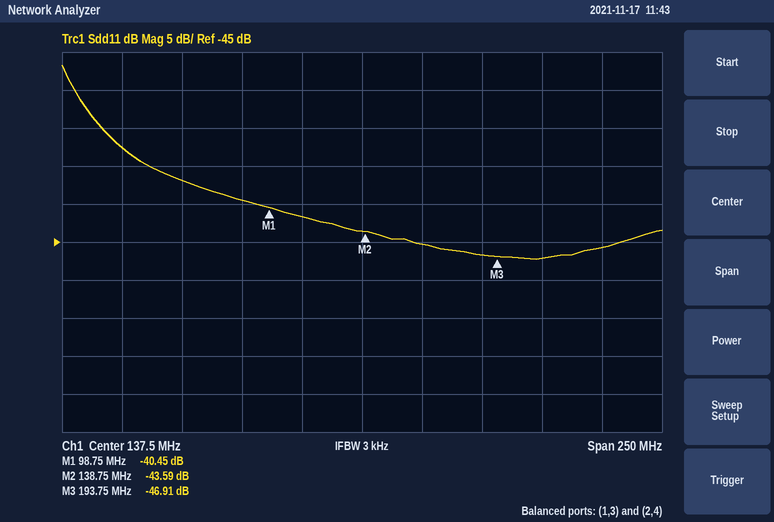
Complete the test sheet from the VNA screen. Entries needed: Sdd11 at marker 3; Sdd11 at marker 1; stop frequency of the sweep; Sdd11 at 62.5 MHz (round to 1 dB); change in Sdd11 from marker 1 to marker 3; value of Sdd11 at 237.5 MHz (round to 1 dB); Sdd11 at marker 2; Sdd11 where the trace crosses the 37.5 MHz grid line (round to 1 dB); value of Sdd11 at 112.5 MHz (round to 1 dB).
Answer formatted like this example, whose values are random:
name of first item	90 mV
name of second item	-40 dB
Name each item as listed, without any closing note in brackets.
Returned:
Sdd11 at marker 3	-46.91 dB
Sdd11 at marker 1	-40.45 dB
stop frequency of the sweep	262.5 MHz
Sdd11 at 62.5 MHz	-37 dB
change in Sdd11 from marker 1 to marker 3	-6.46 dB
value of Sdd11 at 237.5 MHz	-46 dB
Sdd11 at marker 2	-43.59 dB
Sdd11 where the trace crosses the 37.5 MHz grid line	-33 dB
value of Sdd11 at 112.5 MHz	-42 dB
